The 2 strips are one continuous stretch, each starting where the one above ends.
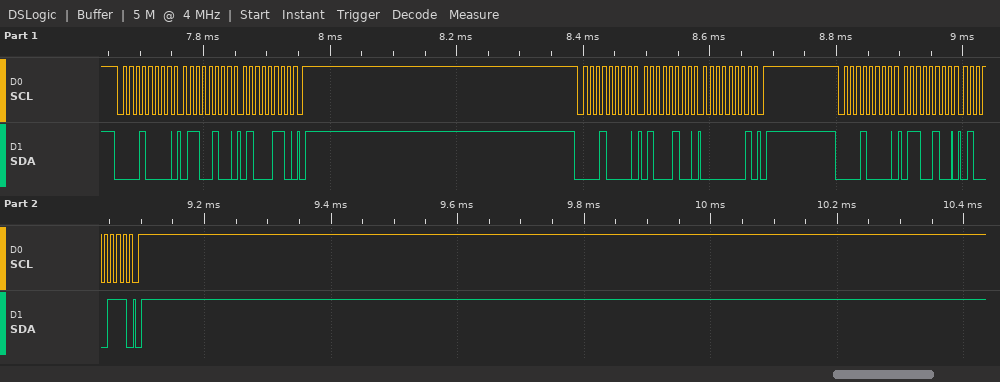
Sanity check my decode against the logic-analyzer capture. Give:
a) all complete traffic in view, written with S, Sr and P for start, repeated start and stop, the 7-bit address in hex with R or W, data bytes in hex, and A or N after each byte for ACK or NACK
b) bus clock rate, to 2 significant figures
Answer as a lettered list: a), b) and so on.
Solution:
a) S 08W A 64 A 46 A P S 08W A 44 A 01 A P S 08W A 64 A 47 A P
b) 100 kHz
